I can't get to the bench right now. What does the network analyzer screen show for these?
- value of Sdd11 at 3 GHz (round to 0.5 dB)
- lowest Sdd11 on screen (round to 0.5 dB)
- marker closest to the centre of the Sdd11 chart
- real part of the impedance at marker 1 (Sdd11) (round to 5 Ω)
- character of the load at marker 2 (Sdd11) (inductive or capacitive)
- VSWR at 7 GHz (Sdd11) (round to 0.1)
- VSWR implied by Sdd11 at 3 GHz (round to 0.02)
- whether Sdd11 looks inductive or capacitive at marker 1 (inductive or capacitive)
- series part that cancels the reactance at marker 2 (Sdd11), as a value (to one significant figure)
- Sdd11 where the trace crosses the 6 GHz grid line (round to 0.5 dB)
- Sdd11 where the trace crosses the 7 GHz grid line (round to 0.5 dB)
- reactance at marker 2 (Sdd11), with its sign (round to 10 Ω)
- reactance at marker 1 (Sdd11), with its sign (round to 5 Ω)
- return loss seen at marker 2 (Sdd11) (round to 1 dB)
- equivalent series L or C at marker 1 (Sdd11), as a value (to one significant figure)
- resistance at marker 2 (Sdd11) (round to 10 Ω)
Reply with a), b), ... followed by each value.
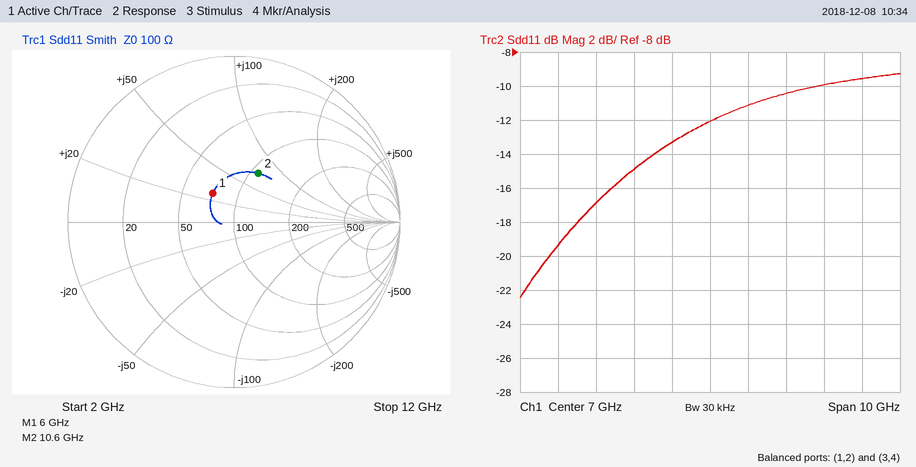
a) -19.5 dB
b) -22.5 dB
c) marker 1
d) 75 Ω
e) inductive
f) 1.7
g) 1.24
h) inductive
i) 200 fF
j) -13.5 dB
k) -12.0 dB
l) +70 Ω
m) +25 Ω
n) 10 dB
o) 700 pH
p) 110 Ω
